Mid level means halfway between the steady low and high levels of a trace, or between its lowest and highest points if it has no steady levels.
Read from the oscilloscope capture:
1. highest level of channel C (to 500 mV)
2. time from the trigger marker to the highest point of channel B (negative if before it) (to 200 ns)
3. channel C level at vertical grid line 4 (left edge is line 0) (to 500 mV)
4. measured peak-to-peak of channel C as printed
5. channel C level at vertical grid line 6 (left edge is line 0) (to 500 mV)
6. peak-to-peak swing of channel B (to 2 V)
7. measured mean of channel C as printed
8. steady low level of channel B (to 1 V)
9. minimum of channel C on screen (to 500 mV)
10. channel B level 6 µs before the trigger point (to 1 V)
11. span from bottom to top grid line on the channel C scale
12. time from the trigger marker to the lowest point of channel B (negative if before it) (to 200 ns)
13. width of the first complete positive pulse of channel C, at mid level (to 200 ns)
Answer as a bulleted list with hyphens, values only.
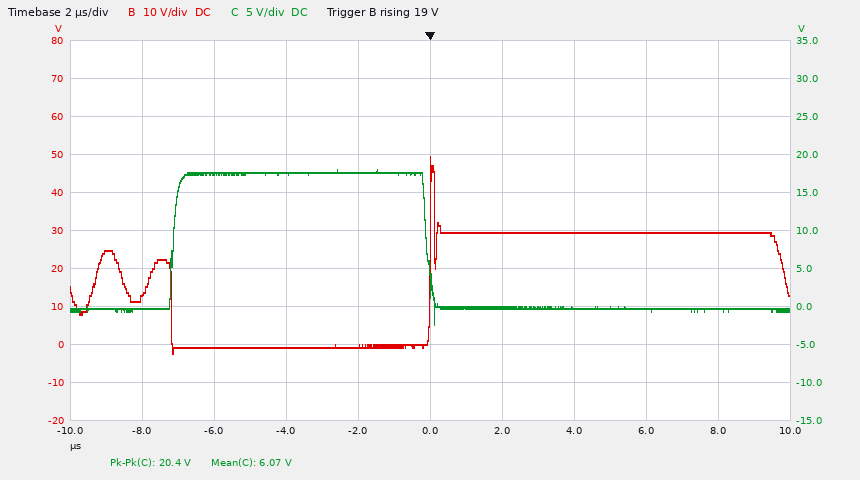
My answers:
- 18.0 V
- 0.0 µs
- 17.5 V
- 20.4 V
- 0.0 V
- 52 V
- 6.07 V
- -1 V
- -2.5 V
- -1 V
- 50 V
- -7.2 µs
- 7.0 µs
